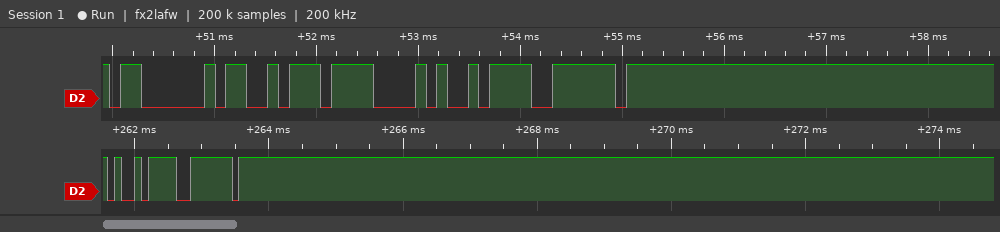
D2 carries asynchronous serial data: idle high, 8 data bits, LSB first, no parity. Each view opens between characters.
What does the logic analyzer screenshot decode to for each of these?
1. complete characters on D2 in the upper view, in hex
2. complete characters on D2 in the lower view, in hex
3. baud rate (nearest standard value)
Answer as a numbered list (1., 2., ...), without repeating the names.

1. 03, D3, 0F, E9, 7E
2. E9, 7E
3. 9600 baud
